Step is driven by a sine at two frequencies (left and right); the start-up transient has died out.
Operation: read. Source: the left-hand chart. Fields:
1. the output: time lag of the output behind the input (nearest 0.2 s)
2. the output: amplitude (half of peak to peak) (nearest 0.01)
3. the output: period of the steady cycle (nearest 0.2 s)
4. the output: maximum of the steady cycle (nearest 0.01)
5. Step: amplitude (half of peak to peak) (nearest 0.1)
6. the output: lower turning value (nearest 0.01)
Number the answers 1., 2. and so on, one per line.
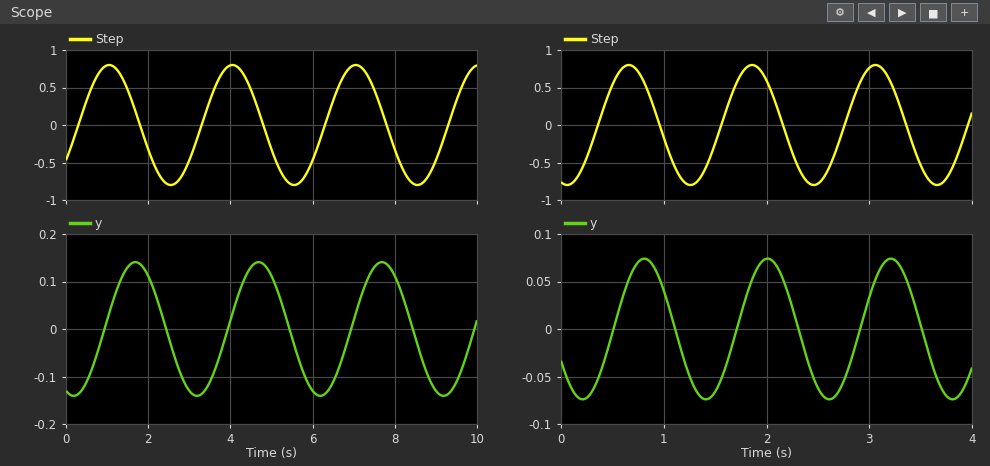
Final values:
1. 0.6 s
2. 0.14
3. 3.0 s
4. 0.14
5. 0.8
6. -0.14
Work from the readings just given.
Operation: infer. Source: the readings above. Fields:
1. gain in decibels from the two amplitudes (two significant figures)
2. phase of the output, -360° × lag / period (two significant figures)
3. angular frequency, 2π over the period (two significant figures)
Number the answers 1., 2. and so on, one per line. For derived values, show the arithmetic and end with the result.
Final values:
1. 20 log10(0.14 / 0.8) = -15 dB
2. -360 × 0.6 / 3 = -72°
3. 2π / 3 = 2.1 rad/s
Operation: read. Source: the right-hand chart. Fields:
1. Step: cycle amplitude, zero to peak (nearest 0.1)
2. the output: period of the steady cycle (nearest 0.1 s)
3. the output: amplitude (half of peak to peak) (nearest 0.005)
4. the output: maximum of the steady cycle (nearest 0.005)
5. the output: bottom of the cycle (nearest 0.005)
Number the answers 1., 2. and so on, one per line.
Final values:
1. 0.8
2. 1.2 s
3. 0.075
4. 0.075
5. -0.075
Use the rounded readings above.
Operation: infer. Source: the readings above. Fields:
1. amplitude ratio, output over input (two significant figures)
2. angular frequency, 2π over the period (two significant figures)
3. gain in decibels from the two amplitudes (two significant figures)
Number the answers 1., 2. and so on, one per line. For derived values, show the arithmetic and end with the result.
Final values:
1. 0.075 / 0.8 = 0.094
2. 2π / 1.2 = 5.2 rad/s
3. 20 log10(0.075 / 0.8) = -21 dB
